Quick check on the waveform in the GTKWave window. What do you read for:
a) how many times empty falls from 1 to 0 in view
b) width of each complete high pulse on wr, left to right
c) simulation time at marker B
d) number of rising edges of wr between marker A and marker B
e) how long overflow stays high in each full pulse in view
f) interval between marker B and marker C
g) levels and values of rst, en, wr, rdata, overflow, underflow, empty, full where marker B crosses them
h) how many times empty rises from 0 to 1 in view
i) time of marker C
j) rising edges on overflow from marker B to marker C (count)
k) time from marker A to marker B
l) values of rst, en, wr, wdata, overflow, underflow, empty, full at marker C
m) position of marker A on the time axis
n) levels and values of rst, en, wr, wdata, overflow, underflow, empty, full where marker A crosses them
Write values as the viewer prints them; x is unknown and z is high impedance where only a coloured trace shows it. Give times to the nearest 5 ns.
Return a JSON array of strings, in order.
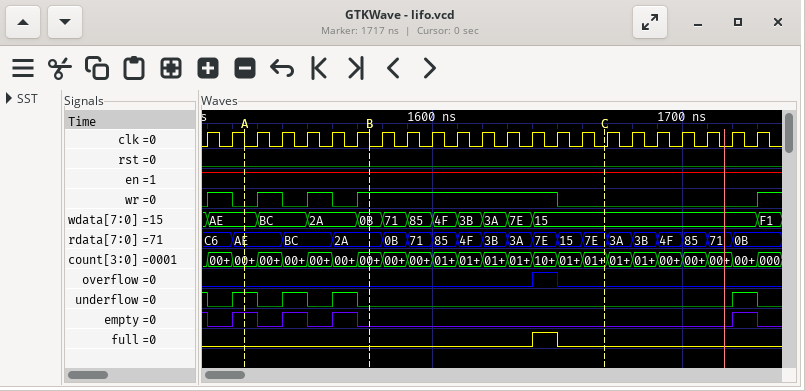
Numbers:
["5", "10 ns, 10 ns, 10 ns, 80 ns", "1575 ns", "3", "10 ns", "95 ns", "rst=0, en=1, wr=1, rdata=2A, overflow=0, underflow=0, empty=0, full=0", "4", "1670 ns", "1", "50 ns", "rst=0, en=1, wr=0, wdata=15, overflow=0, underflow=0, empty=0, full=0", "1525 ns", "rst=0, en=1, wr=0, wdata=AE, overflow=0, underflow=1, empty=1, full=0"]
